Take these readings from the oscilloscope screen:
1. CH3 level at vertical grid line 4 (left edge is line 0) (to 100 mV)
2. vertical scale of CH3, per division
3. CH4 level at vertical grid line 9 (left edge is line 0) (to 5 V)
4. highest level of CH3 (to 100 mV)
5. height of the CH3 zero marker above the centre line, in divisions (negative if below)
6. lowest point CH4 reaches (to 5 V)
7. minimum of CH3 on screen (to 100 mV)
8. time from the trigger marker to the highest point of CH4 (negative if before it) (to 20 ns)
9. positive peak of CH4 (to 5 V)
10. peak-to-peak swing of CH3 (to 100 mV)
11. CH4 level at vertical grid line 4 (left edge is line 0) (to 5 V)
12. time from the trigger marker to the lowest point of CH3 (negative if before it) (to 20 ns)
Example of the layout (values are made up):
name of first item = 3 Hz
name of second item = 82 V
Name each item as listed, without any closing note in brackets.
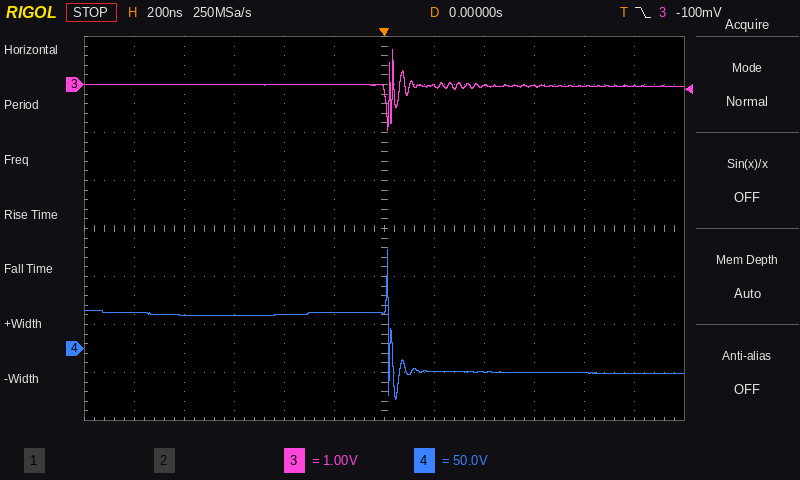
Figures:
CH3 level at vertical grid line 4 (left edge is line 0) = 0.0 V
vertical scale of CH3, per division = 1 V
CH4 level at vertical grid line 9 (left edge is line 0) = -25 V
highest level of CH3 = 700 mV
height of the CH3 zero marker above the centre line, in divisions = +3.0 div
lowest point CH4 reaches = -55 V
minimum of CH3 on screen = -1.0 V
time from the trigger marker to the highest point of CH4 (negative if before it) = +20 ns
positive peak of CH4 = 105 V
peak-to-peak swing of CH3 = 1.7 V
CH4 level at vertical grid line 4 (left edge is line 0) = 35 V
time from the trigger marker to the lowest point of CH3 (negative if before it) = +20 ns
